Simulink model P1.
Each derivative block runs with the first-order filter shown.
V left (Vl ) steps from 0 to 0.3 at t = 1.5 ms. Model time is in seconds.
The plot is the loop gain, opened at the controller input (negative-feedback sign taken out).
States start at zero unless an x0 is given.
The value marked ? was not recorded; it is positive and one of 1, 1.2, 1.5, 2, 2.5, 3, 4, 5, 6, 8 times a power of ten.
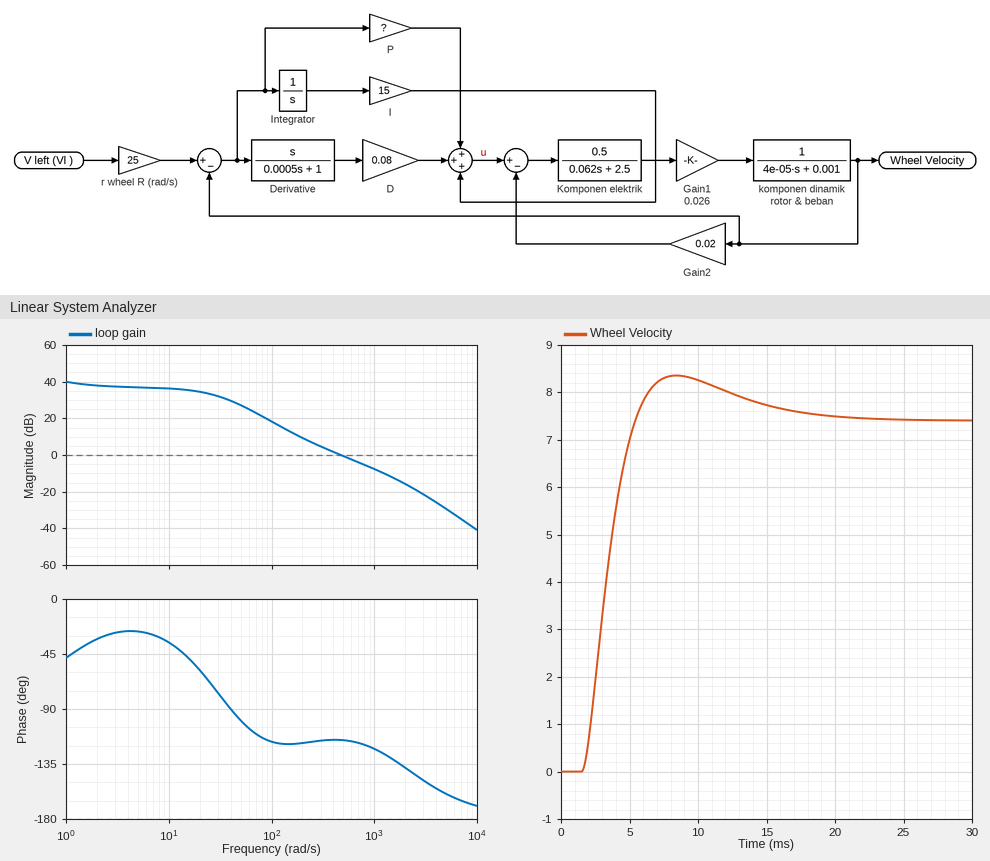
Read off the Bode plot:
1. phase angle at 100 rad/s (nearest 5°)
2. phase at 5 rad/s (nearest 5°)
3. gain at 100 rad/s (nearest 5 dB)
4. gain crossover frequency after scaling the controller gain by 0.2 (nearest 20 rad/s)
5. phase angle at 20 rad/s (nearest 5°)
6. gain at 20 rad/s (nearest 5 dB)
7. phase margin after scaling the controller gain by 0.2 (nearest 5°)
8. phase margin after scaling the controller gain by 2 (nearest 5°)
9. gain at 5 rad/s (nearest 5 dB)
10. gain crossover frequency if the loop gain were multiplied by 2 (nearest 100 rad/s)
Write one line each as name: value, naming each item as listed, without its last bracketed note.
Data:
phase angle at 100 rad/s: -115°
phase at 5 rad/s: -25°
gain at 100 rad/s: 20 dB
gain crossover frequency after scaling the controller gain by 0.2: 140 rad/s
phase angle at 20 rad/s: -60°
gain at 20 rad/s: 35 dB
phase margin after scaling the controller gain by 0.2: 60°
phase margin after scaling the controller gain by 2: 60°
gain at 5 rad/s: 35 dB
gain crossover frequency if the loop gain were multiplied by 2: 900 rad/s
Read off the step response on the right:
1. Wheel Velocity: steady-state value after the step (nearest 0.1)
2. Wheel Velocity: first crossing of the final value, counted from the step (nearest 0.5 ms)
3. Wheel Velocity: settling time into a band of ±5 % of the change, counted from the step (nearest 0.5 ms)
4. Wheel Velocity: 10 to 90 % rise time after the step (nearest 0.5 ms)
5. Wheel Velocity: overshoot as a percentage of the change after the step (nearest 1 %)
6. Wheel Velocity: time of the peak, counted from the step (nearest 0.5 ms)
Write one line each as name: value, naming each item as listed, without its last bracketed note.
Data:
Wheel Velocity: steady-state value after the step: 7.4
Wheel Velocity: first crossing of the final value, counted from the step: 4.0 ms
Wheel Velocity: settling time into a band of ±5 % of the change, counted from the step: 13.0 ms
Wheel Velocity: 10 to 90 % rise time after the step: 2.5 ms
Wheel Velocity: overshoot as a percentage of the change after the step: 13 %
Wheel Velocity: time of the peak, counted from the step: 7.0 ms
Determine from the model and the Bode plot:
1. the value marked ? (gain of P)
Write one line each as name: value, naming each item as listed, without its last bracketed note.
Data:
the value marked ?: 15
